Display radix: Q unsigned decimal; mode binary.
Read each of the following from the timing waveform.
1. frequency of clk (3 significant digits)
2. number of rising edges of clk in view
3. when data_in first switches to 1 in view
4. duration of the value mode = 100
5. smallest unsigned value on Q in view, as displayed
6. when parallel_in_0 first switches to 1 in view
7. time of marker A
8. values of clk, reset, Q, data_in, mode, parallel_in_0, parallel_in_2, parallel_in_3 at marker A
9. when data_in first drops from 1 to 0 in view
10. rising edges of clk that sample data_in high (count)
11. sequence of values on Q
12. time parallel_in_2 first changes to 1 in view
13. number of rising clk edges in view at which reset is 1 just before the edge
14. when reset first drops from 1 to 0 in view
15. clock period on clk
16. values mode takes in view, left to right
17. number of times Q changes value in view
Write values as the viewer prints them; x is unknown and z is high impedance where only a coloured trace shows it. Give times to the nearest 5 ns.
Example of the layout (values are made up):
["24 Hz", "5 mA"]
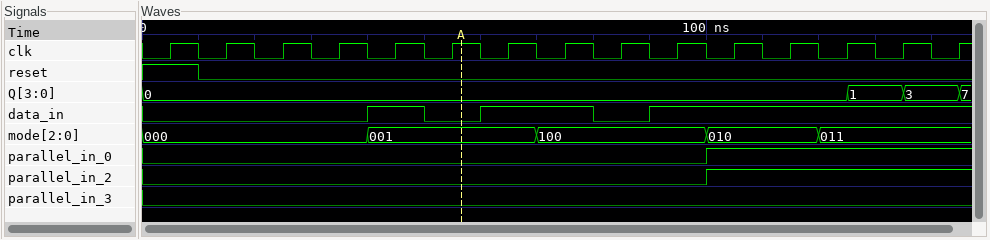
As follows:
["100 MHz", "15", "40 ns", "30 ns", "0", "100 ns", "55 ns", "clk=1, reset=0, Q=0, data_in=0, mode=001, parallel_in_0=0, parallel_in_2=0, parallel_in_3=0", "50 ns", "9", "0, 1, 3, 7", "100 ns", "1", "10 ns", "10 ns", "000, 001, 100, 010, 011", "3"]
